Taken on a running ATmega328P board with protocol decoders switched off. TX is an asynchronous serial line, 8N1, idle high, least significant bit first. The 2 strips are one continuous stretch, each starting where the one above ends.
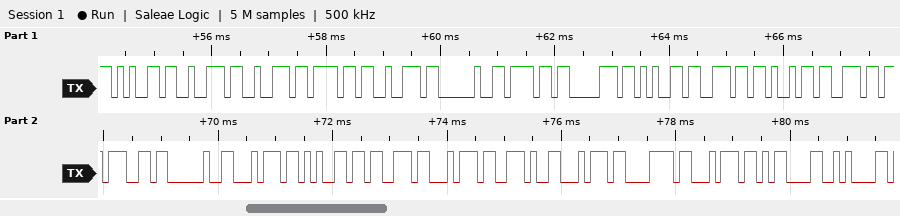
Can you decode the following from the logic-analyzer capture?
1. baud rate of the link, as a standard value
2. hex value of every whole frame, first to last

9600 baud
65 72 72 6F 72 20 6F 70 65 6E 69 6E 67 20 74 65 73 74 2E 74 78 74 0D 0A
